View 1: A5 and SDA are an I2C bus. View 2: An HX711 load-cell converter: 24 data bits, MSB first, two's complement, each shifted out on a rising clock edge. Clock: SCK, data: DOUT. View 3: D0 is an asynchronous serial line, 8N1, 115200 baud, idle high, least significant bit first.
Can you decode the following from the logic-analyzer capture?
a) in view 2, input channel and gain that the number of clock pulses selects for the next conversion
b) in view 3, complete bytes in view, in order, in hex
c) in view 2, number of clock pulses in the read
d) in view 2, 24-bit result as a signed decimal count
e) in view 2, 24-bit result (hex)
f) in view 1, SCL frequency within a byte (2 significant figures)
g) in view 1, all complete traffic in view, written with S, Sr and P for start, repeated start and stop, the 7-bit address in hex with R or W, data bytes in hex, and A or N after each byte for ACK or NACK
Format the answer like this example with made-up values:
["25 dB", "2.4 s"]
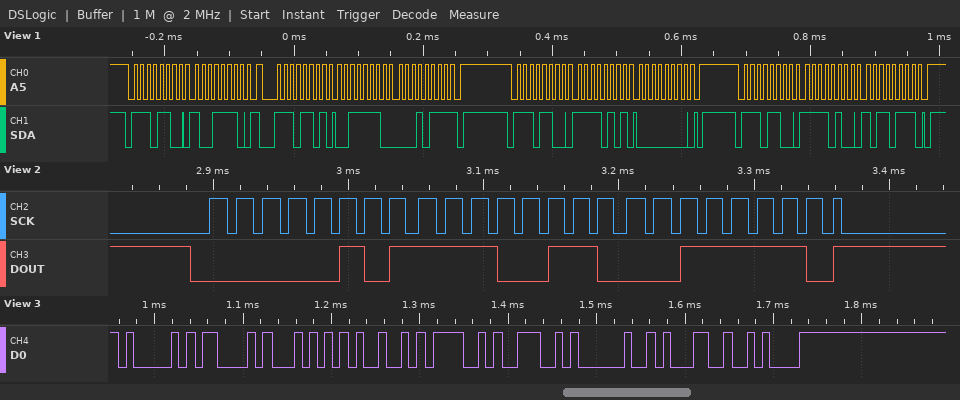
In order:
["channel A, gain 128", "0x41 0x43 0x54 0x49 0x4F 0x4E 0x20 0x31 0x0A", "25", "386622", "0x05E63E", "100 kHz", "S 76W A 9E A Sr 76R A 3E A 17 N P S 76W A F5 A 00 A P S 76W A F4 A B7 A P"]
